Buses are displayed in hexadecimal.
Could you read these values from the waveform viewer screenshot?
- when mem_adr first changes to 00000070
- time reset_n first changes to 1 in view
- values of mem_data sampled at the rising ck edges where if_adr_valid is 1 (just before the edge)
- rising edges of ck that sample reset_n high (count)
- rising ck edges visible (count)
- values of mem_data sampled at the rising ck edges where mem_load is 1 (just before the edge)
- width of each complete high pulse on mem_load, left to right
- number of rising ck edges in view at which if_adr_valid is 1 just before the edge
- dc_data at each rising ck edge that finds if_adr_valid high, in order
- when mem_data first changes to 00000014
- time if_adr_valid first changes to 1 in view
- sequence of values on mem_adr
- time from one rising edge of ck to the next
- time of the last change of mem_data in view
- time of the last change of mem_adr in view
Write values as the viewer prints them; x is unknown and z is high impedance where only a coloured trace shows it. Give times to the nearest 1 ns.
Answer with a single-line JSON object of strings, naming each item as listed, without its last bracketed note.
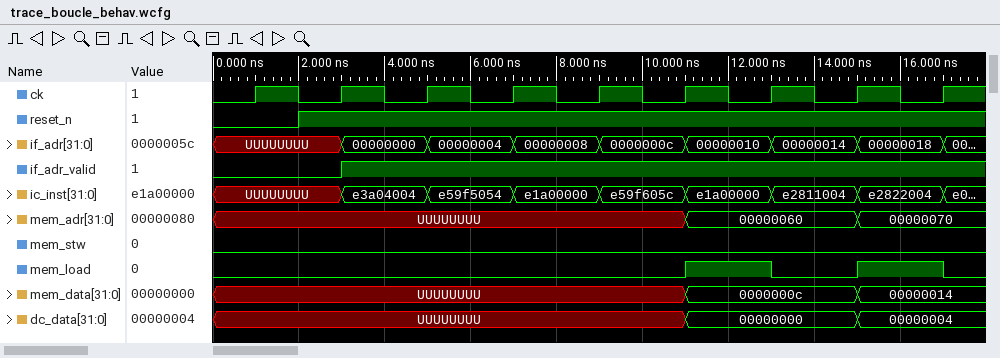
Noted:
{"when mem_adr first changes to 00000070": "15 ns", "time reset_n first changes to 1 in view": "2 ns", "values of mem_data sampled at the rising ck edges where if_adr_valid is 1": "UUUUUUUU, UUUUUUUU, UUUUUUUU, UUUUUUUU, 0000000c, 0000000c, 00000014", "rising edges of ck that sample reset_n high": "8", "rising ck edges visible": "9", "values of mem_data sampled at the rising ck edges where mem_load is 1": "0000000c, 00000014", "width of each complete high pulse on mem_load, left to right": "2 ns, 2 ns", "number of rising ck edges in view at which if_adr_valid is 1 just before the edge": "7", "dc_data at each rising ck edge that finds if_adr_valid high, in order": "UUUUUUUU, UUUUUUUU, UUUUUUUU, UUUUUUUU, 00000000, 00000000, 00000004", "when mem_data first changes to 00000014": "15 ns", "time if_adr_valid first changes to 1 in view": "3 ns", "sequence of values on mem_adr": "UUUUUUUU, 00000060, 00000070", "time from one rising edge of ck to the next": "2 ns", "time of the last change of mem_data in view": "15 ns", "time of the last change of mem_adr in view": "15 ns"}
